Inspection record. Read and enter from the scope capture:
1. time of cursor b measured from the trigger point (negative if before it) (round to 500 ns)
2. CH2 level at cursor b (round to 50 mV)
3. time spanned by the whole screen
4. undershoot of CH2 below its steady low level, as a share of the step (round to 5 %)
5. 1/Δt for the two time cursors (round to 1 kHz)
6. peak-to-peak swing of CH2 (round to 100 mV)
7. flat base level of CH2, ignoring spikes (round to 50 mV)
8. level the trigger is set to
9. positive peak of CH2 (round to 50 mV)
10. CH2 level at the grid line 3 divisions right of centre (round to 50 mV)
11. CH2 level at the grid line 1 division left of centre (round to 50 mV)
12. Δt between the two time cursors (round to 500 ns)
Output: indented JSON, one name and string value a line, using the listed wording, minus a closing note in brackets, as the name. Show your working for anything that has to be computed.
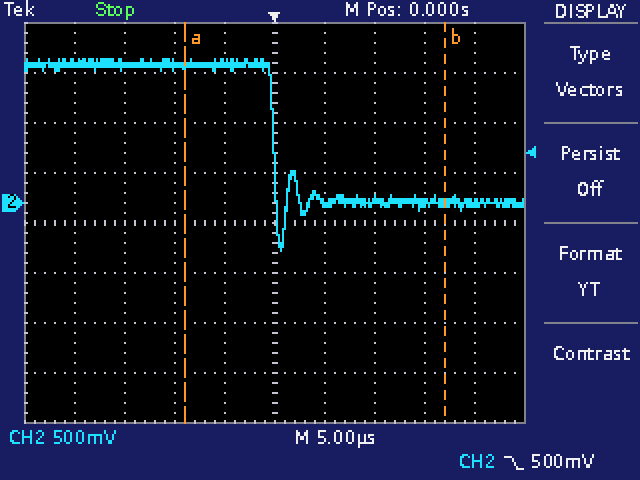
{
  "time of cursor b measured from the trigger point (negative if before it)": "+17.0 µs",
  "CH2 level at cursor b": "0 mV",
  "time spanned by the whole screen": "50 µs",
  "undershoot of CH2 below its steady low level, as a share of the step": "35 %",
  "1/Δt for the two time cursors": "1 / 26.0 µs ≈ 38 kHz",
  "peak-to-peak swing of CH2": "1.90 V",
  "flat base level of CH2, ignoring spikes": "0 mV",
  "level the trigger is set to": "500 mV",
  "positive peak of CH2": "1.45 V",
  "CH2 level at the grid line 3 divisions right of centre": "0 mV",
  "CH2 level at the grid line 1 division left of centre": "1.40 V",
  "Δt between the two time cursors": "26.0 µs"
}
